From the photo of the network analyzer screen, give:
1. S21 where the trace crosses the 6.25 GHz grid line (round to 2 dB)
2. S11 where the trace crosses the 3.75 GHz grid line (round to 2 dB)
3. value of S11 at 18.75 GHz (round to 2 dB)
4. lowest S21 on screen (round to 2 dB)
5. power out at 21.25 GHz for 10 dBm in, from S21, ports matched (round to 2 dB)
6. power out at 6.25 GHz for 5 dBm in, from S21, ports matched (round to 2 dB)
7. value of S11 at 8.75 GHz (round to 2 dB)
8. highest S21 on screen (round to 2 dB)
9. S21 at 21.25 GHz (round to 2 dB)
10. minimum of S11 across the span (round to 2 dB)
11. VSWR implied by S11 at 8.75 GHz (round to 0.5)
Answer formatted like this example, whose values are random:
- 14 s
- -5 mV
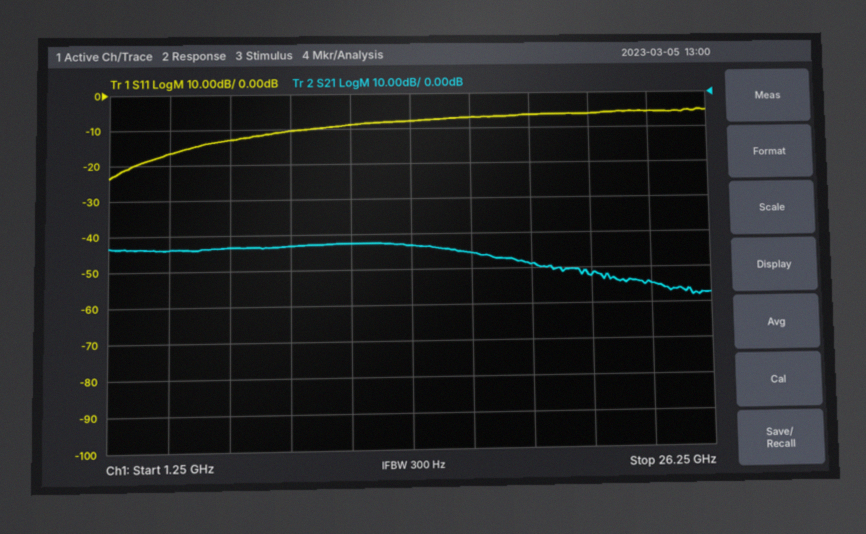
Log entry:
- -44 dB
- -16 dB
- -6 dB
- -58 dB
- -42 dBm
- -38 dBm
- -10 dB
- -42 dB
- -52 dB
- -24 dB
- 2.0
